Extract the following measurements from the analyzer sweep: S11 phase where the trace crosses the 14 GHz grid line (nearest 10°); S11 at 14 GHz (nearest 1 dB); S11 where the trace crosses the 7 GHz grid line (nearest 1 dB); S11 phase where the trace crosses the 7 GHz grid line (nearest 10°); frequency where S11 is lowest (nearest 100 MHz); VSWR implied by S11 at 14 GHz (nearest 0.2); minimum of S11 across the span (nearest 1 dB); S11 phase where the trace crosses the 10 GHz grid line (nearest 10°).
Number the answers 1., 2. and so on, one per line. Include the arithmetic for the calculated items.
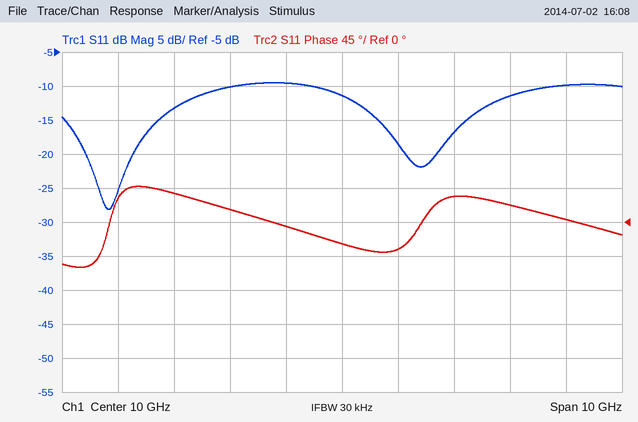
1. 0°
2. -10 dB
3. -13 dB
4. 40°
5. 5.8 GHz
6. |Γ| = 10^(-10/20) = 0.3162; VSWR = (1 + 0.3162)/(1 − 0.3162) ≈ 1.92, so 2.0 to the nearest 0.2
7. -28 dB
8. -30°
